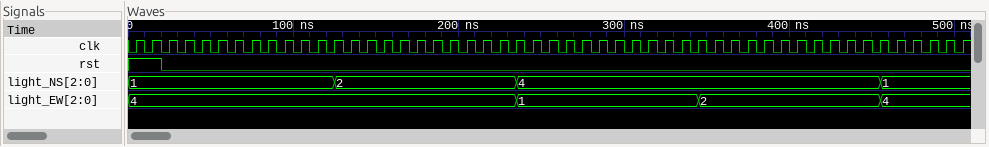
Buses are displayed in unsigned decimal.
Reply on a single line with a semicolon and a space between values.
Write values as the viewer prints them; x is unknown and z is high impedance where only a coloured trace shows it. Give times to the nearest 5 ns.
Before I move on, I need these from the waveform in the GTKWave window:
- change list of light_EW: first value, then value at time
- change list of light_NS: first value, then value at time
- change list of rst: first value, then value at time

4, 1 at 235 ns, 2 at 345 ns, 4 at 455 ns; 1, 2 at 125 ns, 4 at 235 ns, 1 at 455 ns; 1, 0 at 20 ns
